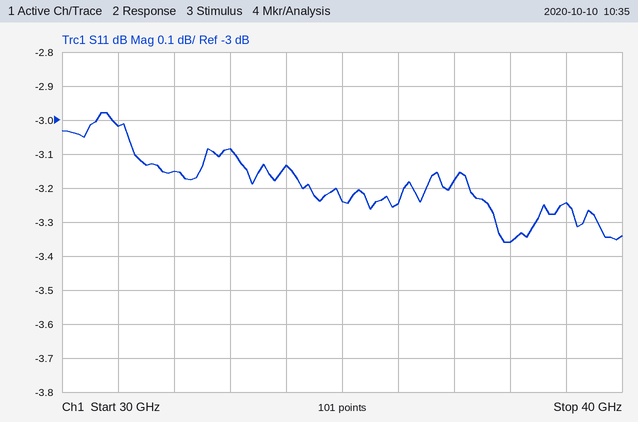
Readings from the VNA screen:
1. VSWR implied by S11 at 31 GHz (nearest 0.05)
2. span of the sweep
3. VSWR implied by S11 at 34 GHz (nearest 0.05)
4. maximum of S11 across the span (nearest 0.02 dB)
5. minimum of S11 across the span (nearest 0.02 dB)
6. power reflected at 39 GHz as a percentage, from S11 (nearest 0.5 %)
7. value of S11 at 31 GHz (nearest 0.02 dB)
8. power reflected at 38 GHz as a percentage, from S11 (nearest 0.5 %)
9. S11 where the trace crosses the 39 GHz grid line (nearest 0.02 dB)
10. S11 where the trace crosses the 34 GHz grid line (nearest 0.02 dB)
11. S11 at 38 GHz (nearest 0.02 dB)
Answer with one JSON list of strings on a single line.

["5.80", "10 GHz", "5.60", "-2.98 dB", "-3.36 dB", "47.5 %", "-3.02 dB", "46.0 %", "-3.24 dB", "-3.14 dB", "-3.36 dB"]
